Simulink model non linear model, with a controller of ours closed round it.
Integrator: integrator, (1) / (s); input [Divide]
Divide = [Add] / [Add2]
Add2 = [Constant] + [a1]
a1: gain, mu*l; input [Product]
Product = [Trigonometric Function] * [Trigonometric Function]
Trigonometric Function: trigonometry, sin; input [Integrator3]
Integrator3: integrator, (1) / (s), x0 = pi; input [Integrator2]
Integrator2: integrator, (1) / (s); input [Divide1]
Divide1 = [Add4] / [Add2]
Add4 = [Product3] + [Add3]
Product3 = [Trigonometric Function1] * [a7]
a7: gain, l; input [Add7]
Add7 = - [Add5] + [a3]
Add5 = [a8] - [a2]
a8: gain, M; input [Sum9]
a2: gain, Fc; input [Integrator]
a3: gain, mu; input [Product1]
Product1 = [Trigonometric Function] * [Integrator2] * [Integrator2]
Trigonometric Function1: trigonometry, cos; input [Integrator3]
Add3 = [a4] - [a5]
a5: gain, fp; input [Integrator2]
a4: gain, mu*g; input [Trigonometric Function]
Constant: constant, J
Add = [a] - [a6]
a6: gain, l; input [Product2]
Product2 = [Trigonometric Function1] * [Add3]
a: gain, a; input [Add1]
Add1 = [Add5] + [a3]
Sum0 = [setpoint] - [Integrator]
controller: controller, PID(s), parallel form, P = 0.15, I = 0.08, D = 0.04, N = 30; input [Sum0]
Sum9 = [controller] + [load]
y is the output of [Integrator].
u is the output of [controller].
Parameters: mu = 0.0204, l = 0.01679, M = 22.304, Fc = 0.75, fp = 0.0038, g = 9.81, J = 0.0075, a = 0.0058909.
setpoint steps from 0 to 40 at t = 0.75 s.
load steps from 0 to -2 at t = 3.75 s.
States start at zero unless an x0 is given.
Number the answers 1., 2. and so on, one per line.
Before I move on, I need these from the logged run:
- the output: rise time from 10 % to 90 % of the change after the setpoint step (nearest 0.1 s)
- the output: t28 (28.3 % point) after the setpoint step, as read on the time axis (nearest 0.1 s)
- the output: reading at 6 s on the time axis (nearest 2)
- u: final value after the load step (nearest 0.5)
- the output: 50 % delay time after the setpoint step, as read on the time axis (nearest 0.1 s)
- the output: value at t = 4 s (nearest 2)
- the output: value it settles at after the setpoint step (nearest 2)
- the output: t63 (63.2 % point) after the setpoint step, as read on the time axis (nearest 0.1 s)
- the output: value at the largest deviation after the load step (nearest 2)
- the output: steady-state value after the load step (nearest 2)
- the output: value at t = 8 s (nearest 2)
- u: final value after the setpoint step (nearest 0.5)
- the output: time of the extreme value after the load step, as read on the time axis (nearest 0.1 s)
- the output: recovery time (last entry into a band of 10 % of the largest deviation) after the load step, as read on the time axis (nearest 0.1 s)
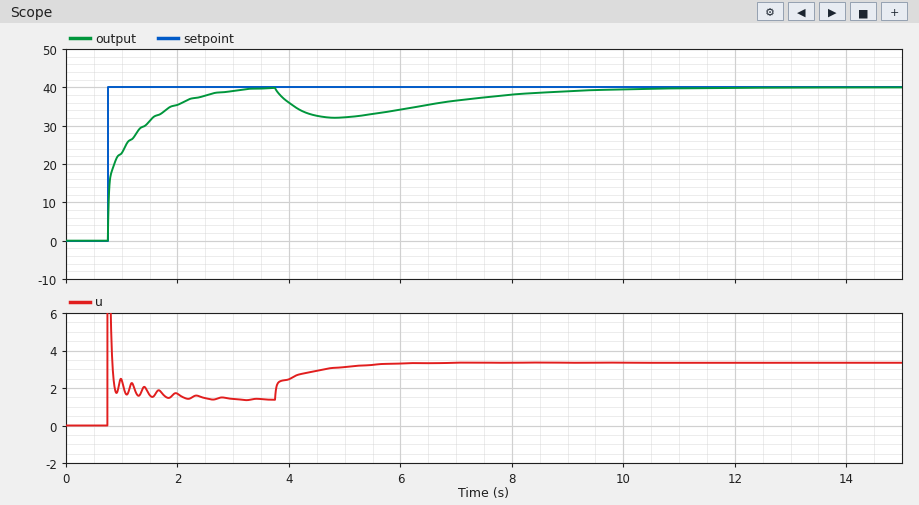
1. 1.3 s
2. 0.8 s
3. 34
4. 3.5
5. 0.9 s
6. 36
7. 40
8. 1.1 s
9. 32
10. 40
11. 38
12. 1.5
13. 4.8 s
14. 9.4 s
